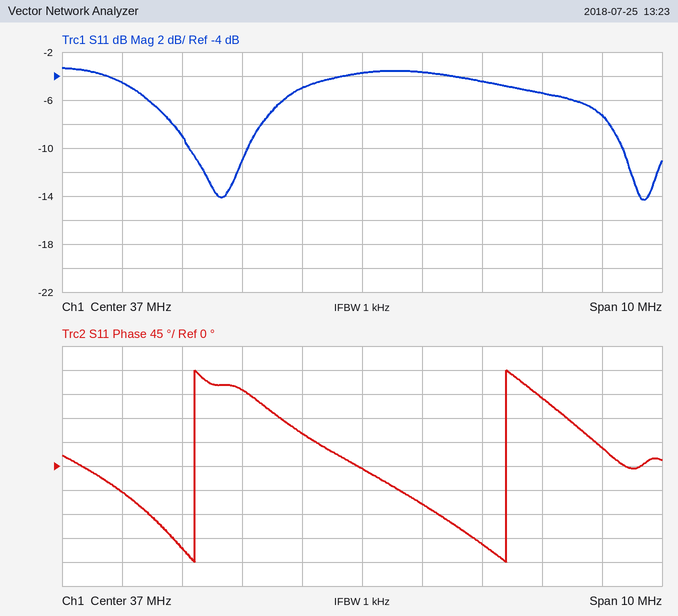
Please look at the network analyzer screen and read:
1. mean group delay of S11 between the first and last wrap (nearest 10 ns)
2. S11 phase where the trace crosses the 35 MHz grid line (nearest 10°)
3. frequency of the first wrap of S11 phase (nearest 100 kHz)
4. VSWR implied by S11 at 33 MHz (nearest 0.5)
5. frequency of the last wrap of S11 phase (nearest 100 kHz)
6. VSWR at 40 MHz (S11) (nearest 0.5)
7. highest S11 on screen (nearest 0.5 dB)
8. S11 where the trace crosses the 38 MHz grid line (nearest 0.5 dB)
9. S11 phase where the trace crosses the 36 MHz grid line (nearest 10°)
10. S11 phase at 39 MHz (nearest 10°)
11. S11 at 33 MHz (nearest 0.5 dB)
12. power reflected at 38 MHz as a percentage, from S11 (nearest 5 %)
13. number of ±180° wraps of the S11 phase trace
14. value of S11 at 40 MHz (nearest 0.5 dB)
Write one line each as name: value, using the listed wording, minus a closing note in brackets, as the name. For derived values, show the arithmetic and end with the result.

mean group delay of S11 between the first and last wrap: 1 cycle / (39.4 MHz − 34.2 MHz) ≈ 192 ns, so 190 ns to the nearest 10 ns
S11 phase where the trace crosses the 35 MHz grid line: 140°
frequency of the first wrap of S11 phase: 34.2 MHz
VSWR implied by S11 at 33 MHz: |Γ| = 10^(-4.5/20) = 0.5957; VSWR = (1 + 0.5957)/(1 − 0.5957) ≈ 4.0
frequency of the last wrap of S11 phase: 39.4 MHz
VSWR at 40 MHz (S11): |Γ| = 10^(-5.5/20) = 0.5309; VSWR = (1 + 0.5309)/(1 − 0.5309) ≈ 3.26, so 3.5 to the nearest 0.5
highest S11 on screen: -3.5 dB
S11 where the trace crosses the 38 MHz grid line: -3.5 dB
S11 phase where the trace crosses the 36 MHz grid line: 60°
S11 phase at 39 MHz: -150°
S11 at 33 MHz: -4.5 dB
power reflected at 38 MHz as a percentage, from S11: 10^(-3.5/10) ≈ 45 %
number of ±180° wraps of the S11 phase trace: 2
value of S11 at 40 MHz: -5.5 dB
